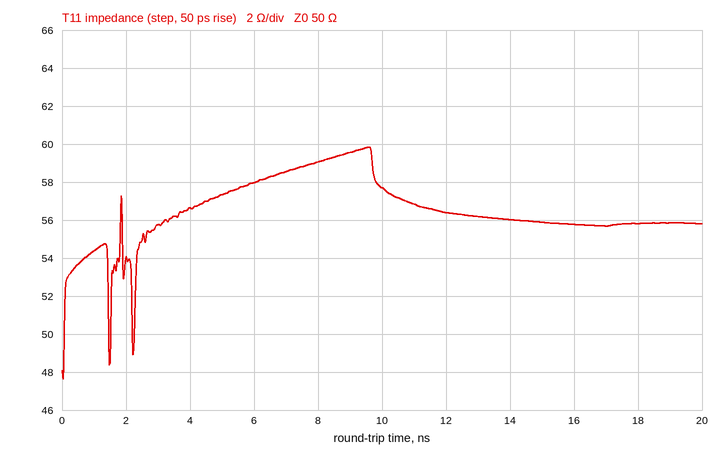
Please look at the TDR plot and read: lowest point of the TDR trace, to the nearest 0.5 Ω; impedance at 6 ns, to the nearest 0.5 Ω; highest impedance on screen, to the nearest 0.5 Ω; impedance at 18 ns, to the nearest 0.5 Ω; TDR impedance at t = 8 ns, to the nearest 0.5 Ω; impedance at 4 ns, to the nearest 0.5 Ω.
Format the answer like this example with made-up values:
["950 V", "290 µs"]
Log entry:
["47.5 Ω", "58.0 Ω", "60.0 Ω", "56.0 Ω", "59.0 Ω", "56.5 Ω"]
